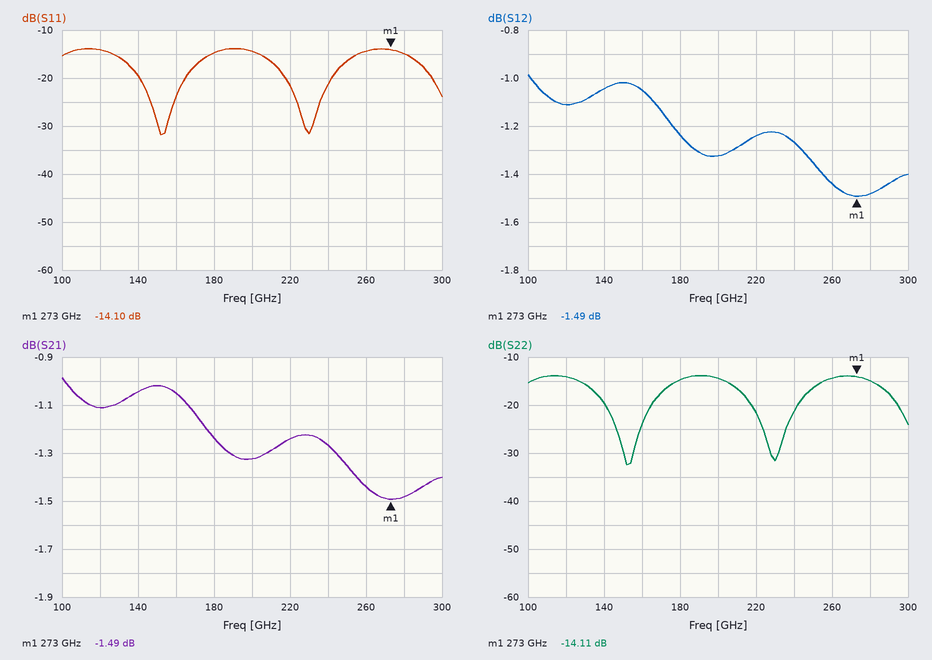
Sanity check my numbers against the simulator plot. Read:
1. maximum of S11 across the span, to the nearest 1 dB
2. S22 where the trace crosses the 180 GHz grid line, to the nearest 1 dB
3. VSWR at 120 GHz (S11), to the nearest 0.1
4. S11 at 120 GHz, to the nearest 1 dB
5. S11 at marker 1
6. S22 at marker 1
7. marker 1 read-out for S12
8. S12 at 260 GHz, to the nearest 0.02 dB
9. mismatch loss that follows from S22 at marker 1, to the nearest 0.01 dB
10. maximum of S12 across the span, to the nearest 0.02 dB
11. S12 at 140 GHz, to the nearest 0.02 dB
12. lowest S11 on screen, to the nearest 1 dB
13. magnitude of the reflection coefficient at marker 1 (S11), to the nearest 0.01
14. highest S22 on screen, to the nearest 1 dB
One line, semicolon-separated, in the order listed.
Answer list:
-14 dB; -15 dB; 1.5; -14 dB; -14.10 dB; -14.11 dB; -1.49 dB; -1.44 dB; 0.17 dB; -0.98 dB; -1.04 dB; -32 dB; 0.20; -14 dB
